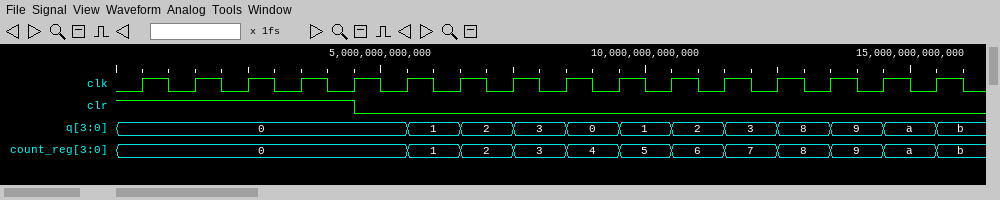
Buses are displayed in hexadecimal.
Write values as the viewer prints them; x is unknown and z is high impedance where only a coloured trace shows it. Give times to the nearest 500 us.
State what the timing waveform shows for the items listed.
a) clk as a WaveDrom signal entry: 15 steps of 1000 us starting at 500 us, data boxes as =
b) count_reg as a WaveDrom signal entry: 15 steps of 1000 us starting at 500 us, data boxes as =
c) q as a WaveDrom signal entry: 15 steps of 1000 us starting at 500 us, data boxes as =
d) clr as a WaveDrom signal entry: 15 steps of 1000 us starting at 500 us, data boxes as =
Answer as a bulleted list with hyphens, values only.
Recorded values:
- {name: 'clk', wave: 'p..............'}
- {name: 'count_reg', wave: '=....==========', data: '0 1 2 3 4 5 6 7 8 9 a'}
- {name: 'q', wave: '=....==========', data: '0 1 2 3 0 1 2 3 8 9 a'}
- {name: 'clr', wave: '1...0..........'}
